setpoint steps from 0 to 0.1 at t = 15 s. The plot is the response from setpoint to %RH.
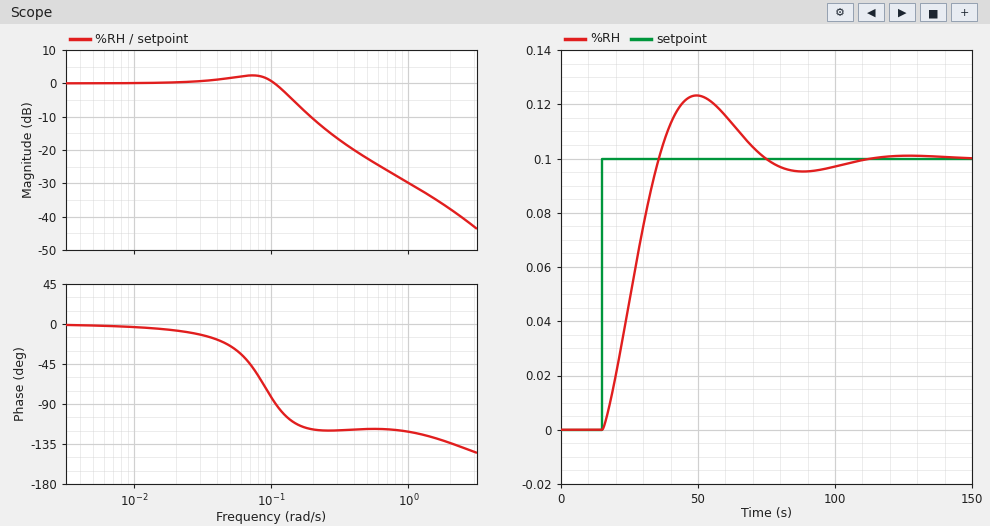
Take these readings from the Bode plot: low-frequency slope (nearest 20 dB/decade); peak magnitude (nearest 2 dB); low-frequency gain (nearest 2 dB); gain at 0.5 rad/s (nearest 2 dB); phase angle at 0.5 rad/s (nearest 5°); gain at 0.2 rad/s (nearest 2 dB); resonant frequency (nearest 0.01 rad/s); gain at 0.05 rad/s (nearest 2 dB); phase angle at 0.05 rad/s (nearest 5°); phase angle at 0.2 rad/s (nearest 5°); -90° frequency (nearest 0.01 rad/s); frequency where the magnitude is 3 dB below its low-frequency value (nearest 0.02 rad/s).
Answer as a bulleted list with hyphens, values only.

- 0 dB/decade
- 2 dB
- 0 dB
- -22 dB
- -120°
- -10 dB
- 0.07 rad/s
- 2 dB
- -25°
- -120°
- 0.11 rad/s
- 0.12 rad/s
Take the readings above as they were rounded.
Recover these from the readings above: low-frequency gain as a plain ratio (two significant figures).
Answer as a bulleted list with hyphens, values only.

- 1.0
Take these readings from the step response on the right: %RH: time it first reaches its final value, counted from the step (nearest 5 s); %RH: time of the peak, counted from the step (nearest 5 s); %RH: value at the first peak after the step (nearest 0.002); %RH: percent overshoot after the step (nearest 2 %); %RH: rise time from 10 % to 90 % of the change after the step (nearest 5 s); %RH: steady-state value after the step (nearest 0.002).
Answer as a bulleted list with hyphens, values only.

- 20 s
- 35 s
- 0.124
- 24 %
- 15 s
- 0.100
